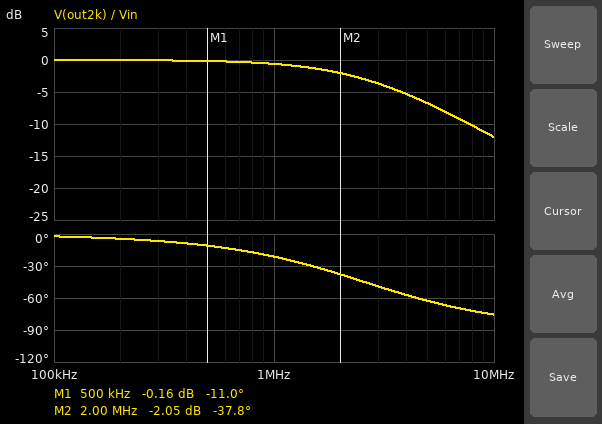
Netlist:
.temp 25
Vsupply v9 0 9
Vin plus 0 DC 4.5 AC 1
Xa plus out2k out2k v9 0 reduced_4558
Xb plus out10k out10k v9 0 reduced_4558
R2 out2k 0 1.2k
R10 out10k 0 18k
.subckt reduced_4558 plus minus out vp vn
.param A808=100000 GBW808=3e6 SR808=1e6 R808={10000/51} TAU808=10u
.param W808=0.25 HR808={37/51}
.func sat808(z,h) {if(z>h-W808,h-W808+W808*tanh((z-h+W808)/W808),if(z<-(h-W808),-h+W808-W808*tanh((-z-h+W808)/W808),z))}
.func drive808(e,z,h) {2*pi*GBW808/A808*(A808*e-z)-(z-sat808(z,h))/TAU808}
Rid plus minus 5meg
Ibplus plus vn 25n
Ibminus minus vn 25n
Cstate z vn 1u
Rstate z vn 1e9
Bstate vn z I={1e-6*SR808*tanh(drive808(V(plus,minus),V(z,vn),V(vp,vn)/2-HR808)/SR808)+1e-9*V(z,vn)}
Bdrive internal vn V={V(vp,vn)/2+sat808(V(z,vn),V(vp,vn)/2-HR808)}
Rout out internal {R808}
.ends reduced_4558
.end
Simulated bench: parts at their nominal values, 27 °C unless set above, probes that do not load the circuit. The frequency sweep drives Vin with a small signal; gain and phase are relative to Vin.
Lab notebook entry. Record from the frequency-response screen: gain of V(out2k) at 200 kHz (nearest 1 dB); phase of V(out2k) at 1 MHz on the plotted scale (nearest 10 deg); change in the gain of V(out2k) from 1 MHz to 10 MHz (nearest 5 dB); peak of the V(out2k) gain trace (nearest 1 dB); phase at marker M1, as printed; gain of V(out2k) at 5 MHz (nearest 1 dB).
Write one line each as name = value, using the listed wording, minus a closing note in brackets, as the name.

gain of V(out2k) at 200 kHz = 0 dB
phase of V(out2k) at 1 MHz on the plotted scale = -20 deg
change in the gain of V(out2k) from 1 MHz to 10 MHz = -10 dB
peak of the V(out2k) gain trace = 0 dB
phase at marker M1, as printed = -11.0 deg
gain of V(out2k) at 5 MHz = -7 dB
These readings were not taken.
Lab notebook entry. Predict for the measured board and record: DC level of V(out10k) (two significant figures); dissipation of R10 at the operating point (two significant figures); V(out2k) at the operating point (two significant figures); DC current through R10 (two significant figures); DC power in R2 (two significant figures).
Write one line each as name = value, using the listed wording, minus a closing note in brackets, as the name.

DC level of V(out10k) = 4.5 V
dissipation of R10 at the operating point = 1.1 mW
V(out2k) at the operating point = 4.5 V
DC current through R10 = 250 µA
DC power in R2 = 17 mW
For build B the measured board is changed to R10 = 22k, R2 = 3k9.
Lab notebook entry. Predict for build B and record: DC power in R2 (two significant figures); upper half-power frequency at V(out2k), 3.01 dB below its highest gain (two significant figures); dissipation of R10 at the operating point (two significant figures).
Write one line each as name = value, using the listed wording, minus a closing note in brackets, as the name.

DC power in R2 = 5.2 mW
upper half-power frequency at V(out2k), 3.01 dB below its highest gain = 2.9 MHz
dissipation of R10 at the operating point = 920 µW
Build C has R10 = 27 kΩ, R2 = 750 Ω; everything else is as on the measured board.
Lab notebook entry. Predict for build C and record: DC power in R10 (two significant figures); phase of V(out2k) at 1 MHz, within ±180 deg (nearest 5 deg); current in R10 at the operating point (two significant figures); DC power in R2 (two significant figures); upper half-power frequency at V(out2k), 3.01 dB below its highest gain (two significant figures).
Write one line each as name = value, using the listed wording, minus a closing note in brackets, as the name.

DC power in R10 = 750 µW
phase of V(out2k) at 1 MHz, within ±180 deg = -25 deg
current in R10 at the operating point = 170 µA
DC power in R2 = 27 mW
upper half-power frequency at V(out2k), 3.01 dB below its highest gain = 2.4 MHz
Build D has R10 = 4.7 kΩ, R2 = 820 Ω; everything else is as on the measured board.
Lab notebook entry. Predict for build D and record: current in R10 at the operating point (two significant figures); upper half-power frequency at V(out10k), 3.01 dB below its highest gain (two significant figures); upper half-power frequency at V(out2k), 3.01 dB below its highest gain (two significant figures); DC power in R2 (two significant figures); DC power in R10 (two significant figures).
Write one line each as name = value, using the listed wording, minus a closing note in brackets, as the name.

current in R10 at the operating point = 960 µA
upper half-power frequency at V(out10k), 3.01 dB below its highest gain = 2.9 MHz
upper half-power frequency at V(out2k), 3.01 dB below its highest gain = 2.4 MHz
DC power in R2 = 25 mW
DC power in R10 = 4.3 mW
